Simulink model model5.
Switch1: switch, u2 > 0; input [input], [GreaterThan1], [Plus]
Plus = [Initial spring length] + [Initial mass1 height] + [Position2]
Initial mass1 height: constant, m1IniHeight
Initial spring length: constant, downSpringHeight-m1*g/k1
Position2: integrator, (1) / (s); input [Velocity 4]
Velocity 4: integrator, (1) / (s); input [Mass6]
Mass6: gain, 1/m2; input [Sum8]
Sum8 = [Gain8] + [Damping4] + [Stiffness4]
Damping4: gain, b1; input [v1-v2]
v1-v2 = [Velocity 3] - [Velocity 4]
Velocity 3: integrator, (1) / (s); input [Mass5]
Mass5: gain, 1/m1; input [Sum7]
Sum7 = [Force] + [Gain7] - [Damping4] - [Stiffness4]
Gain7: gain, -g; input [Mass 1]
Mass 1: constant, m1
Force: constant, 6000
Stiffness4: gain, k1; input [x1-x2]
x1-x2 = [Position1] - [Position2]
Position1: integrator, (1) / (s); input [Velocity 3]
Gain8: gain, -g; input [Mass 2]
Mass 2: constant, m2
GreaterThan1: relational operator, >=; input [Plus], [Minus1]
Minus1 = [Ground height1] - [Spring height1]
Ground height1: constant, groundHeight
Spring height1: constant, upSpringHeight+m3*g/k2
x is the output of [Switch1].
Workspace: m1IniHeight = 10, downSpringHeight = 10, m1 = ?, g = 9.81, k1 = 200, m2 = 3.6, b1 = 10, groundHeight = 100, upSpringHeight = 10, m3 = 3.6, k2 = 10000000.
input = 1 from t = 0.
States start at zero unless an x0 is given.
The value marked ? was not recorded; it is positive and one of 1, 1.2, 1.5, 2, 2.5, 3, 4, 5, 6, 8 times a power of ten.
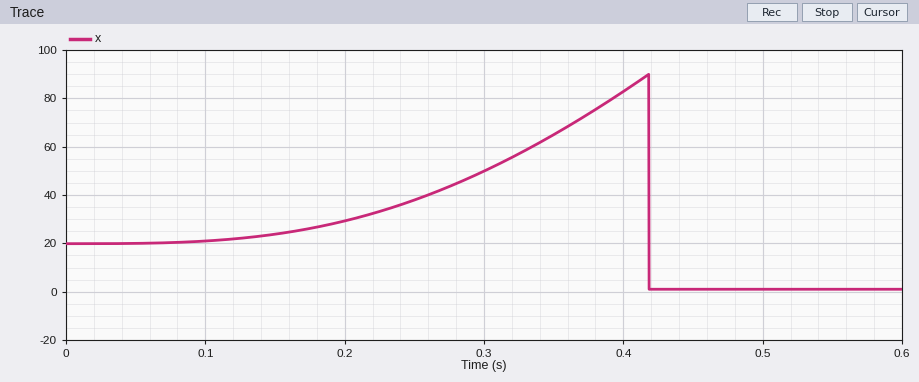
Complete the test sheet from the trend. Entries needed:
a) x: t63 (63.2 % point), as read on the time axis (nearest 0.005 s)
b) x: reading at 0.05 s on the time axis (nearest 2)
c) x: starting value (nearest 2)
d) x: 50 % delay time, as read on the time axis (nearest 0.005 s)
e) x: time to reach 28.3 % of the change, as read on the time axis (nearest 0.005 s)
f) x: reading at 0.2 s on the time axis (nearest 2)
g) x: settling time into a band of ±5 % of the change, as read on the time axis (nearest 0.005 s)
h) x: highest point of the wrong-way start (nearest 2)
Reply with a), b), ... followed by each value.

a) 0.420 s
b) 20
c) 20
d) 0.420 s
e) 0.420 s
f) 30
g) 0.420 s
h) 90
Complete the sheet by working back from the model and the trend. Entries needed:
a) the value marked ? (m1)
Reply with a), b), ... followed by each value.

a) 3
